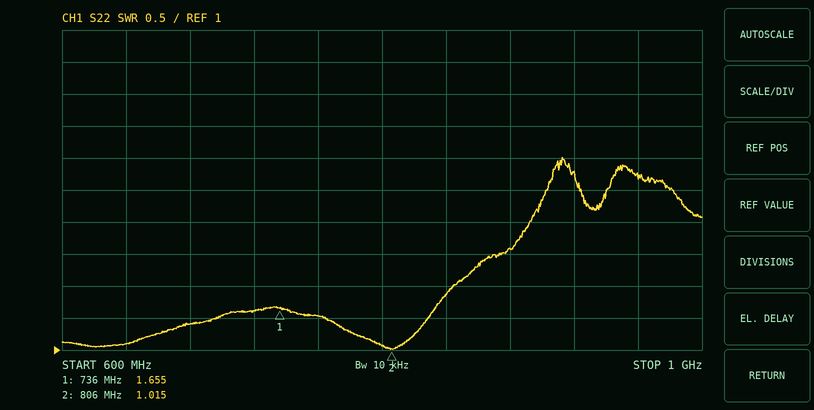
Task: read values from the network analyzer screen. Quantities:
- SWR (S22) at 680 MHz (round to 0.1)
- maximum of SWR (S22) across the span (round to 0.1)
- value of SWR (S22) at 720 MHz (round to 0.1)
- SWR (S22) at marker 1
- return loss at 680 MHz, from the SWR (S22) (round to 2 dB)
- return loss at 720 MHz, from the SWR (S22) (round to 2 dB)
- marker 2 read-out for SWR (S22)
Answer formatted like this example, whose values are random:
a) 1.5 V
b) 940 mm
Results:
a) 1.4
b) 4.0
c) 1.6
d) 1.655
e) 16 dB
f) 12 dB
g) 1.015
